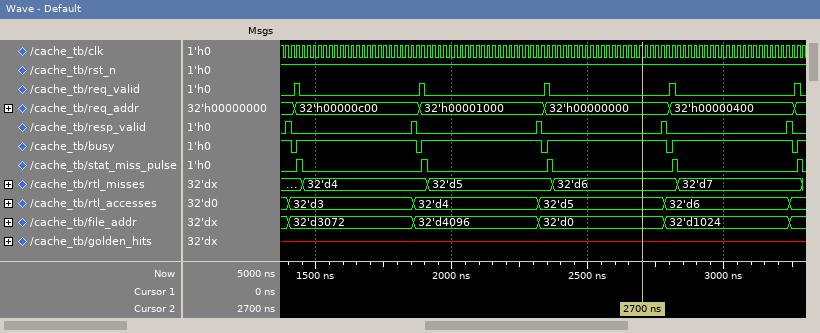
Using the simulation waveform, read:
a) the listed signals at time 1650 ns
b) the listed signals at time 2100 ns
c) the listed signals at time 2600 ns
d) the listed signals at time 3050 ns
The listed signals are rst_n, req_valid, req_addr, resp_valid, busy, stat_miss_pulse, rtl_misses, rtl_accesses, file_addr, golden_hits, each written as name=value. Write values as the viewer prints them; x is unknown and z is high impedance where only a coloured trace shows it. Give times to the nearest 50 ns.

rst_n=1, req_valid=0, req_addr=32'h00000c00, resp_valid=0, busy=1, stat_miss_pulse=0, rtl_misses=32'd4, rtl_accesses=32'd3, file_addr=32'd3072, golden_hits=x
rst_n=1, req_valid=0, req_addr=32'h00001000, resp_valid=0, busy=1, stat_miss_pulse=0, rtl_misses=32'd5, rtl_accesses=32'd4, file_addr=32'd4096, golden_hits=x
rst_n=1, req_valid=0, req_addr=32'h00000000, resp_valid=0, busy=1, stat_miss_pulse=0, rtl_misses=32'd6, rtl_accesses=32'd5, file_addr=32'd0, golden_hits=x
rst_n=1, req_valid=0, req_addr=32'h00000400, resp_valid=0, busy=1, stat_miss_pulse=0, rtl_misses=32'd7, rtl_accesses=32'd6, file_addr=32'd1024, golden_hits=x
